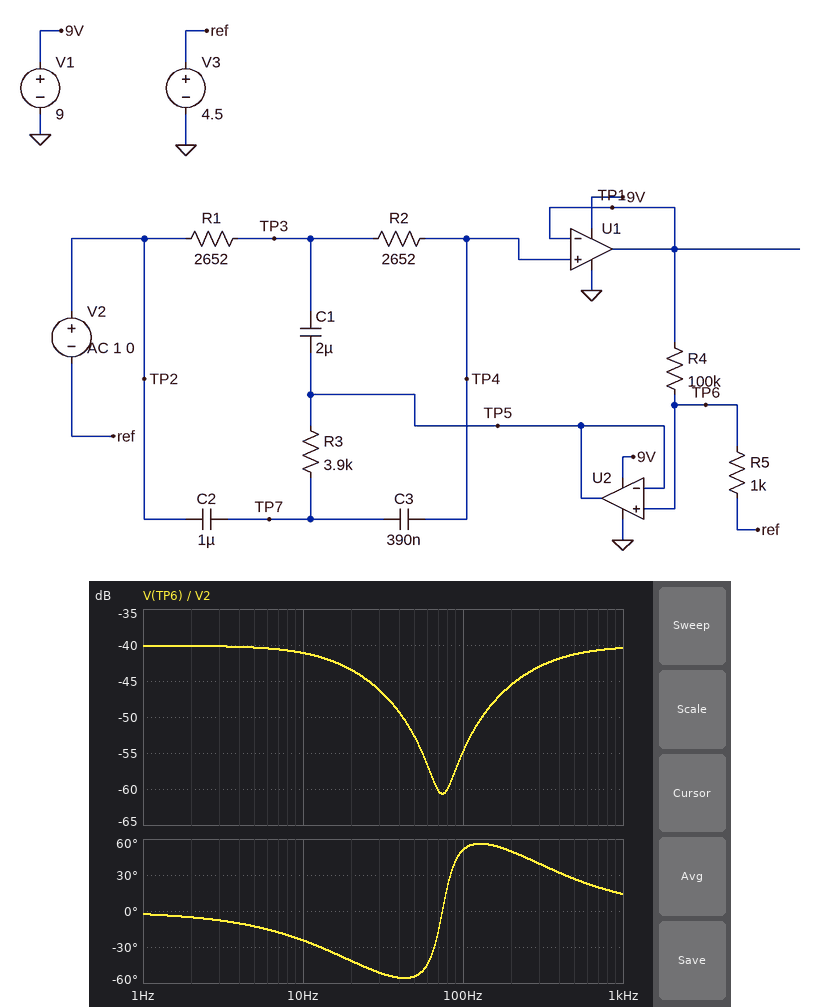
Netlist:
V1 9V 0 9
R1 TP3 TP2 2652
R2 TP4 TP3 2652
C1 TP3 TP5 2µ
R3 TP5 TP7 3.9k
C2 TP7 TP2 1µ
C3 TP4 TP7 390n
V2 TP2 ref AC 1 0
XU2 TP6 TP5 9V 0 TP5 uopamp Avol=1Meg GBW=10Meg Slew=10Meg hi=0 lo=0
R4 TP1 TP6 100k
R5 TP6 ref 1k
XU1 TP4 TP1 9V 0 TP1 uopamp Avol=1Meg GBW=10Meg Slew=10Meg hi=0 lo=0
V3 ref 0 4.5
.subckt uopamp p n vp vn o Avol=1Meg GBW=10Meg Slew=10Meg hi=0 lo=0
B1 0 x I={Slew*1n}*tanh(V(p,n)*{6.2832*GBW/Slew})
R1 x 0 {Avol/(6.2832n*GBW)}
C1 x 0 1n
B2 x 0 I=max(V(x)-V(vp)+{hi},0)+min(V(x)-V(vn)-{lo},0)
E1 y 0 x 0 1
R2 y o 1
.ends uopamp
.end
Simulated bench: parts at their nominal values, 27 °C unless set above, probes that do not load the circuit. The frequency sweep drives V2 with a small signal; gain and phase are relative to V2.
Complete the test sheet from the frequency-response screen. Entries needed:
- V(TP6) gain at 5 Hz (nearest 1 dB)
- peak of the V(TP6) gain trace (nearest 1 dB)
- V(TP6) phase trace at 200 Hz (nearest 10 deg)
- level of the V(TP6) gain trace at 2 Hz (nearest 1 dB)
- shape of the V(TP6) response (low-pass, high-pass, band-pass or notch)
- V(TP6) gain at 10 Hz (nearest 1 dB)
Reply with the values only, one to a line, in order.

-40 dB
-40 dB
50 deg
-40 dB
notch
-41 dB
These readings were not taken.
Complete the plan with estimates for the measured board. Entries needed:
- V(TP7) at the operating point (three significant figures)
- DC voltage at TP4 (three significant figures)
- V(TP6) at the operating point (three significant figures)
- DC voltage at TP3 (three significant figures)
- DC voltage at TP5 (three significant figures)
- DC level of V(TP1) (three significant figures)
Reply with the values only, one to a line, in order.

4.50 V
4.50 V
4.50 V
4.50 V
4.50 V
4.50 V
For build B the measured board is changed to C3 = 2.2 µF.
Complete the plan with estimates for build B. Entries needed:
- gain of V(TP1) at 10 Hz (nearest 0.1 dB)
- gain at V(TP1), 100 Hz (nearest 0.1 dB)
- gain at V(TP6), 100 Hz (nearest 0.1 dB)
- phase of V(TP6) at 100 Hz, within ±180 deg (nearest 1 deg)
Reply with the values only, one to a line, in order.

-4.5 dB
-6.1 dB
-46.2 dB
41 deg
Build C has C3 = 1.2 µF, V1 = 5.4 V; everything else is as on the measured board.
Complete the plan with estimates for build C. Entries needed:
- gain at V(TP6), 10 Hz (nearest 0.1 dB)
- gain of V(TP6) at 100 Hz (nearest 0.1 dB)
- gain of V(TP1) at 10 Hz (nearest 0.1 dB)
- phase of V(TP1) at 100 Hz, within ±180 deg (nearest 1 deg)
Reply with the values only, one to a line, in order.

-42.7 dB
-47.6 dB
-2.6 dB
45 deg
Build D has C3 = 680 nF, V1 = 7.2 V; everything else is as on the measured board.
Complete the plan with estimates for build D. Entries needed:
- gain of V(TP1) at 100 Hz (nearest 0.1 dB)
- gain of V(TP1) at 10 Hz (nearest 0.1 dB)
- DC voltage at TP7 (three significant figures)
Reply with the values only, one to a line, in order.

-10.1 dB
-1.6 dB
4.50 V
